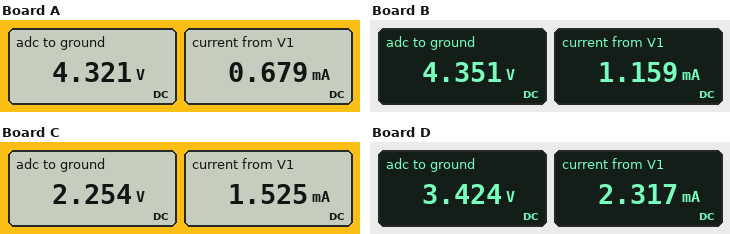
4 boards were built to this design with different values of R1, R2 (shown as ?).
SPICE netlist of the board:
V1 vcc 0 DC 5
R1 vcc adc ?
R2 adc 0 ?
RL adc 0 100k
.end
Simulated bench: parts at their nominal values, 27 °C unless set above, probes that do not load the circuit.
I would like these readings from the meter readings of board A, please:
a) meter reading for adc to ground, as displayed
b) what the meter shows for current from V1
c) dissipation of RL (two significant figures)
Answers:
4.321 V
0.679 mA
190 µW
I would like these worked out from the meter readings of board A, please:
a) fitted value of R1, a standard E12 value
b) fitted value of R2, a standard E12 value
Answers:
1 kΩ
6.8 kΩ
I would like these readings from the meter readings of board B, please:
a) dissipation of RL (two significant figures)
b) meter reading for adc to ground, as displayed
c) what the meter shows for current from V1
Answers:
190 µW
4.351 V
1.159 mA
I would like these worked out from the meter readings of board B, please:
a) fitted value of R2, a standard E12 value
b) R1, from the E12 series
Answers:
3.9 kΩ
560 Ω
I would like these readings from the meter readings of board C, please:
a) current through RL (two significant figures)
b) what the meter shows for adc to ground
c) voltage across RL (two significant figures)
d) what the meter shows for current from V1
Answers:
23 µA
2.254 V
2.3 V
1.525 mA
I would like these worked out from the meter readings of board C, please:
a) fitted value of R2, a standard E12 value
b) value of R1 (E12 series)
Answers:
1.5 kΩ
1.8 kΩ
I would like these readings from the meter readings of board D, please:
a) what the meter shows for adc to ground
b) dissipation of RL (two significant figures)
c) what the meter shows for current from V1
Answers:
3.424 V
120 µW
2.317 mA
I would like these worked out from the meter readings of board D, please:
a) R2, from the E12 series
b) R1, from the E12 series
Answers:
1.5 kΩ
680 Ω
